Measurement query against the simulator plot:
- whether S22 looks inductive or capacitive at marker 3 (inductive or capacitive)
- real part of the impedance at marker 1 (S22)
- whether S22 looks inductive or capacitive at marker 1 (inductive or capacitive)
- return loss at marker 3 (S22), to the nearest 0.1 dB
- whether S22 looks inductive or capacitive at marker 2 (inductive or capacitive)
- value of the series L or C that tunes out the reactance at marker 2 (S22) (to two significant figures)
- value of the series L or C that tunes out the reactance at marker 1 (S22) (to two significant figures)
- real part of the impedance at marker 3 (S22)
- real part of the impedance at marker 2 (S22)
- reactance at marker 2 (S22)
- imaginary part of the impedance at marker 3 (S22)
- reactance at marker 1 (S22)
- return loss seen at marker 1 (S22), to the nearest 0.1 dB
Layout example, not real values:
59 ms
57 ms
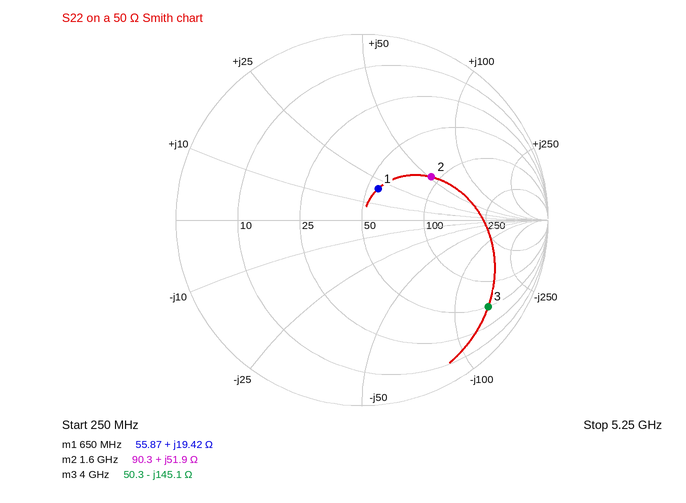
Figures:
capacitive
55.87 Ω
inductive
1.7 dB
inductive
1.9 pF
13 pF
50.3 Ω
90.3 Ω
+51.9 Ω
-145.1 Ω
+19.42 Ω
14.5 dB
